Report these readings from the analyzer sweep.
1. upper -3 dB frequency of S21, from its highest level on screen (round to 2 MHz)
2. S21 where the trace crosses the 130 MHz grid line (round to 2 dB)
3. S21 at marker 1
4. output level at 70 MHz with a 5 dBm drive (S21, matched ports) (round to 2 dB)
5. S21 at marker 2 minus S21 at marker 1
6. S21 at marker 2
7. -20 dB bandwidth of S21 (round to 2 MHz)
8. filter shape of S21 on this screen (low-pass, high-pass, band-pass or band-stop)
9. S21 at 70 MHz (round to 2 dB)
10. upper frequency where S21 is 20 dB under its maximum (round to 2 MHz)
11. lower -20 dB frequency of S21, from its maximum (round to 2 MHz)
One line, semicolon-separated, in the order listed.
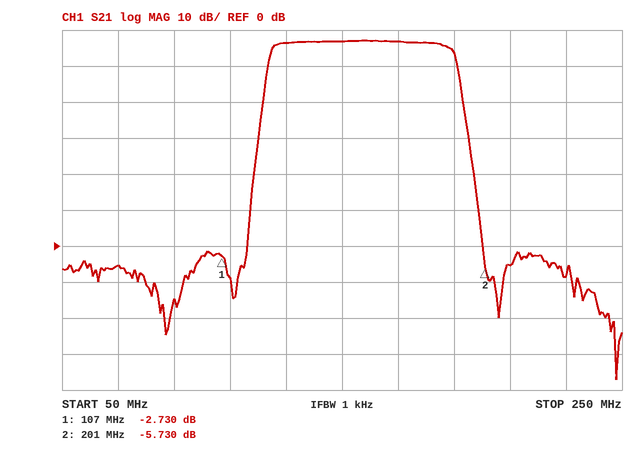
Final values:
190 MHz; 56 dB; -2.730 dB; 0 dBm; -3.000 dB; -5.730 dB; 72 MHz; band-pass; -6 dB; 194 MHz; 122 MHz
